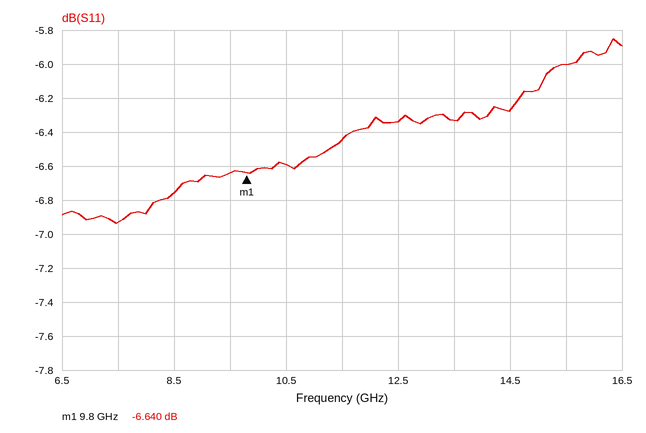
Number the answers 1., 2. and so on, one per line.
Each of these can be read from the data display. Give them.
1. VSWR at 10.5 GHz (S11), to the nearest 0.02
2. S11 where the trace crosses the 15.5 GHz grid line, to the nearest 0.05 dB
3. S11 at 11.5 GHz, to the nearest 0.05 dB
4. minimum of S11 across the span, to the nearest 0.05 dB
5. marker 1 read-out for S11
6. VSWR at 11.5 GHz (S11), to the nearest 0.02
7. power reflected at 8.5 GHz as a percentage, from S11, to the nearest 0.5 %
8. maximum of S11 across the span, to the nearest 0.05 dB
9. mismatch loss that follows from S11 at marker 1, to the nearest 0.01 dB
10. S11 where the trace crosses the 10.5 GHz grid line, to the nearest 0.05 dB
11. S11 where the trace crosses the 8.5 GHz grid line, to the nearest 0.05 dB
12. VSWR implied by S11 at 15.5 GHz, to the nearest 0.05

1. 2.76
2. -6.00 dB
3. -6.45 dB
4. -6.95 dB
5. -6.640 dB
6. 2.82
7. 21.0 %
8. -5.85 dB
9. 1.06 dB
10. -6.60 dB
11. -6.75 dB
12. 3.00
